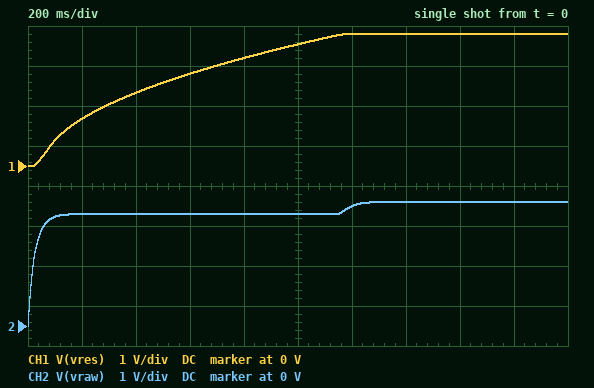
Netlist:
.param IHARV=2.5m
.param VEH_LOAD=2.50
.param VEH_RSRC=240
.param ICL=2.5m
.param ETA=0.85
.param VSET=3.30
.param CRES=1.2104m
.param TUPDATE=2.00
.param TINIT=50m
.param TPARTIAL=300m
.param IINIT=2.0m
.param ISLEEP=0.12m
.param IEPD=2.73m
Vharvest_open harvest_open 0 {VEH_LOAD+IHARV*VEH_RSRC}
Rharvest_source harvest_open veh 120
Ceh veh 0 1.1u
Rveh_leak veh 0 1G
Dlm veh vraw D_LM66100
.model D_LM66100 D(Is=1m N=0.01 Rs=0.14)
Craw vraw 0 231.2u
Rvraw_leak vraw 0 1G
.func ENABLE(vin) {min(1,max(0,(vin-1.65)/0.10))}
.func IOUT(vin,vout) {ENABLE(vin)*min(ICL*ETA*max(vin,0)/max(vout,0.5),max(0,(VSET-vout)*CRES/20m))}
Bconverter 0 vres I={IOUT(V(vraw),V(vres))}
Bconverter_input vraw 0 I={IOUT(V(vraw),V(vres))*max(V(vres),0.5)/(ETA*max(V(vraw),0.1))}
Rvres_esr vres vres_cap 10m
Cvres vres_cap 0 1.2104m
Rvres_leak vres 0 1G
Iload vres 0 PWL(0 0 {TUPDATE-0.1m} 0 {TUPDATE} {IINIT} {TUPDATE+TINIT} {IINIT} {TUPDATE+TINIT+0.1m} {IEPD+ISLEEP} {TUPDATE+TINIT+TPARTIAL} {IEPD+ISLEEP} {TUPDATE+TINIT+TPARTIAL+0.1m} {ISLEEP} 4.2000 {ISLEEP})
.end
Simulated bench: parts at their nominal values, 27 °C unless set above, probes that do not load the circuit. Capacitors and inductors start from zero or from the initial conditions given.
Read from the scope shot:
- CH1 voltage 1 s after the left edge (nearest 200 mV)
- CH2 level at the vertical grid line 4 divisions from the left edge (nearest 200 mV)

3.0 V
2.8 V
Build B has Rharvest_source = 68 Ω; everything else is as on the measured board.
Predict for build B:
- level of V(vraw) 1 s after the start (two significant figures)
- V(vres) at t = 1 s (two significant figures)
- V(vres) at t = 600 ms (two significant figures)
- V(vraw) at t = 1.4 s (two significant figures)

2.9 V
3.1 V
2.4 V
3.1 V
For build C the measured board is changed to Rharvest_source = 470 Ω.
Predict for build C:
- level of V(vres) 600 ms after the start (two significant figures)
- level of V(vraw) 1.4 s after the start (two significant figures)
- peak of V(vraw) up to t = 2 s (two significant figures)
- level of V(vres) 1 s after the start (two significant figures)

1.8 V
1.9 V
3.0 V
2.4 V
